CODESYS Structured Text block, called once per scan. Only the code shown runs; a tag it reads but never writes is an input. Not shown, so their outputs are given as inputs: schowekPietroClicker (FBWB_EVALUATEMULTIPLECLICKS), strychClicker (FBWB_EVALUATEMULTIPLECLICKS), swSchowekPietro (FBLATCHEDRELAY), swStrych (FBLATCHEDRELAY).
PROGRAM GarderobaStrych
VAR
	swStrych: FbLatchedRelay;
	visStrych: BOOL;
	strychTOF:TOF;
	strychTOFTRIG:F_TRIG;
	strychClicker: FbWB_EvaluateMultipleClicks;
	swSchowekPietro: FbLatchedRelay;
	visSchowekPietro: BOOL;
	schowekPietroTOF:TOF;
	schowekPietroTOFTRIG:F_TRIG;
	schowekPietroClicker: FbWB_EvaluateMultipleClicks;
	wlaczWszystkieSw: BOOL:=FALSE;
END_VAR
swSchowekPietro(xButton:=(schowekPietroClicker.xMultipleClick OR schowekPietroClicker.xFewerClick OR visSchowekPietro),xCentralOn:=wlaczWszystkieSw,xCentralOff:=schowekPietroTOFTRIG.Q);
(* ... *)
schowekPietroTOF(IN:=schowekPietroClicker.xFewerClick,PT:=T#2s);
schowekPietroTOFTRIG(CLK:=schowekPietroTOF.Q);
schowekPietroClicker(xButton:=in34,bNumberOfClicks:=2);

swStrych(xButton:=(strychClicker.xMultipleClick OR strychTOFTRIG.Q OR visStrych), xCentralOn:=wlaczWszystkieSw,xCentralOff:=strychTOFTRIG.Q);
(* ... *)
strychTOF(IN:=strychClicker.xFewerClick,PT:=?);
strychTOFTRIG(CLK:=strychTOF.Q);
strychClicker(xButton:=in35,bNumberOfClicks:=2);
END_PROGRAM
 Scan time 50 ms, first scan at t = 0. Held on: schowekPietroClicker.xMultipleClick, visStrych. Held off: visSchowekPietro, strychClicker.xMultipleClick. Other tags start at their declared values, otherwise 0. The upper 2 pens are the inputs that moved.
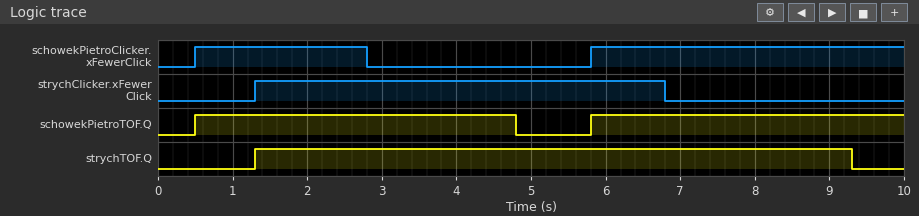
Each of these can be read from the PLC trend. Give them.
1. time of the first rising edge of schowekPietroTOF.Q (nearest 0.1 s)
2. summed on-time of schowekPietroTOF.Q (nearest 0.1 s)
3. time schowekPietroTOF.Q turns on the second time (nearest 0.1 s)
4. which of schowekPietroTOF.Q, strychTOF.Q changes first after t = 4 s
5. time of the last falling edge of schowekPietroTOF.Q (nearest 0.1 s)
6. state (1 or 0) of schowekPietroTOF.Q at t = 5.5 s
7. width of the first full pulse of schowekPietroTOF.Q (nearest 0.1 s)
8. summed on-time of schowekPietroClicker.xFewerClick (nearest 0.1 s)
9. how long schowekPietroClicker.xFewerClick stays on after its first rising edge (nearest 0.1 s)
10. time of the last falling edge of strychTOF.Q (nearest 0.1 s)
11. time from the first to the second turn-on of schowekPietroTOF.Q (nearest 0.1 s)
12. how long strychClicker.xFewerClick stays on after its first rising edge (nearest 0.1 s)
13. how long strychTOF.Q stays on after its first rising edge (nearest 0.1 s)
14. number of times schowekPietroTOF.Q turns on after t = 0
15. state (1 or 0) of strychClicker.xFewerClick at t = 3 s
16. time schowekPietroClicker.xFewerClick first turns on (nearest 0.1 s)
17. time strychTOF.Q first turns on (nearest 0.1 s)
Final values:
0.5 s
8.5 s
5.8 s
schowekPietroTOF.Q
4.8 s
0
4.3 s
6.5 s
2.3 s
9.3 s
5.3 s
5.5 s
8.0 s
2
1
0.5 s
1.3 s
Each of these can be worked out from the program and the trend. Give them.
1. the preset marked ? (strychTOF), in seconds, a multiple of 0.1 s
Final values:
2.5 s
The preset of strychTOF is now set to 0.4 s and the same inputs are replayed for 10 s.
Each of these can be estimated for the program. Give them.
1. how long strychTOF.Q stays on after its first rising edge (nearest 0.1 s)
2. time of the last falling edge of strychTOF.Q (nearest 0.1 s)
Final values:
5.9 s
7.2 s
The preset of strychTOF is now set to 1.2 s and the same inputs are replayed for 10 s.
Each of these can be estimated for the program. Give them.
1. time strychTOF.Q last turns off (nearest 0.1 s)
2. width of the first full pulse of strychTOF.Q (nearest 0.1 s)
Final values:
8.0 s
6.7 s
